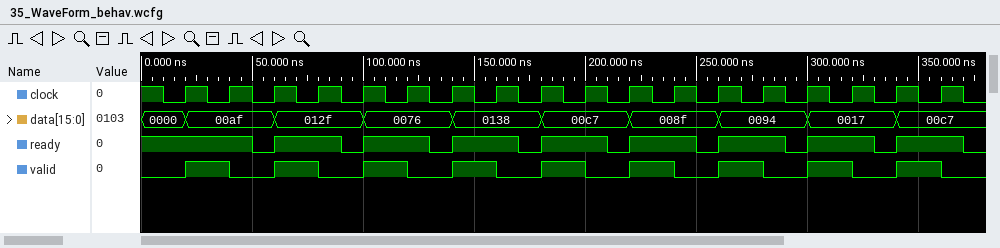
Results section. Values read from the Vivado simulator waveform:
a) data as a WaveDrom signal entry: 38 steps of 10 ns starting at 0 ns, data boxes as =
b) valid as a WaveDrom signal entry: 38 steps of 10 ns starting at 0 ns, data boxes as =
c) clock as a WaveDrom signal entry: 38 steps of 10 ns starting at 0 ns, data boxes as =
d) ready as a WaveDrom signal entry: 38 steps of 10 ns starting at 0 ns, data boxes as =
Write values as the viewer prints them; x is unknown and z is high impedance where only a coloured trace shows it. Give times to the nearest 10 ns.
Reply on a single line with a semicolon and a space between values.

{name: 'data', wave: '=.=...=...=...=...=...=...=...=...=...', data: '0000 00af 012f 0076 0138 00c7 008f 0094 0017 00c7'}; {name: 'valid', wave: '0.1.0.1.0.1.0.1.0.1.0.1.0.1.0.1.0.1.0.'}; {name: 'clock', wave: '10101010101010101010101010101010101010'}; {name: 'ready', wave: '1....01..01..01..01..01..01..01..01..0'}
